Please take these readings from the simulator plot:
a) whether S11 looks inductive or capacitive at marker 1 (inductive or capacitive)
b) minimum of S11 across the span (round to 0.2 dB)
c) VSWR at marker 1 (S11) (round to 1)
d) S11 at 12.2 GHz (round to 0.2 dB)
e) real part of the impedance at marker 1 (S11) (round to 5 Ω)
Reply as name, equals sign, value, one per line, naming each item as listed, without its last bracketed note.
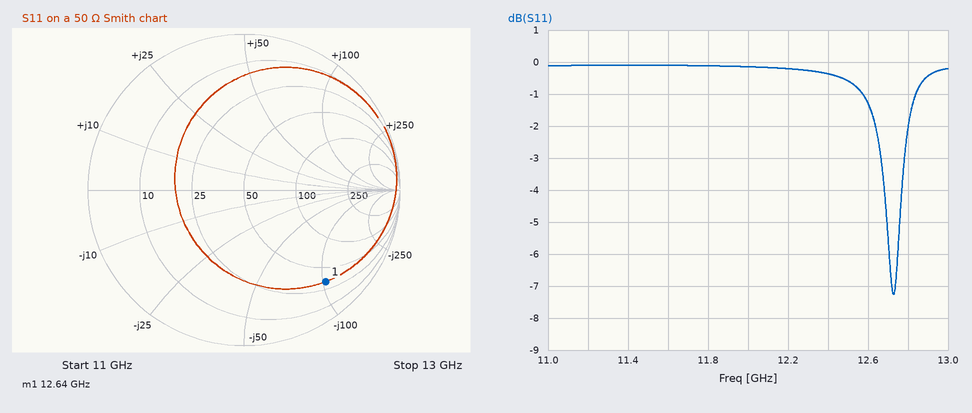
whether S11 looks inductive or capacitive at marker 1 = capacitive
minimum of S11 across the span = -7.2 dB
VSWR at marker 1 (S11) = 8
S11 at 12.2 GHz = -0.2 dB
real part of the impedance at marker 1 (S11) = 35 Ω
